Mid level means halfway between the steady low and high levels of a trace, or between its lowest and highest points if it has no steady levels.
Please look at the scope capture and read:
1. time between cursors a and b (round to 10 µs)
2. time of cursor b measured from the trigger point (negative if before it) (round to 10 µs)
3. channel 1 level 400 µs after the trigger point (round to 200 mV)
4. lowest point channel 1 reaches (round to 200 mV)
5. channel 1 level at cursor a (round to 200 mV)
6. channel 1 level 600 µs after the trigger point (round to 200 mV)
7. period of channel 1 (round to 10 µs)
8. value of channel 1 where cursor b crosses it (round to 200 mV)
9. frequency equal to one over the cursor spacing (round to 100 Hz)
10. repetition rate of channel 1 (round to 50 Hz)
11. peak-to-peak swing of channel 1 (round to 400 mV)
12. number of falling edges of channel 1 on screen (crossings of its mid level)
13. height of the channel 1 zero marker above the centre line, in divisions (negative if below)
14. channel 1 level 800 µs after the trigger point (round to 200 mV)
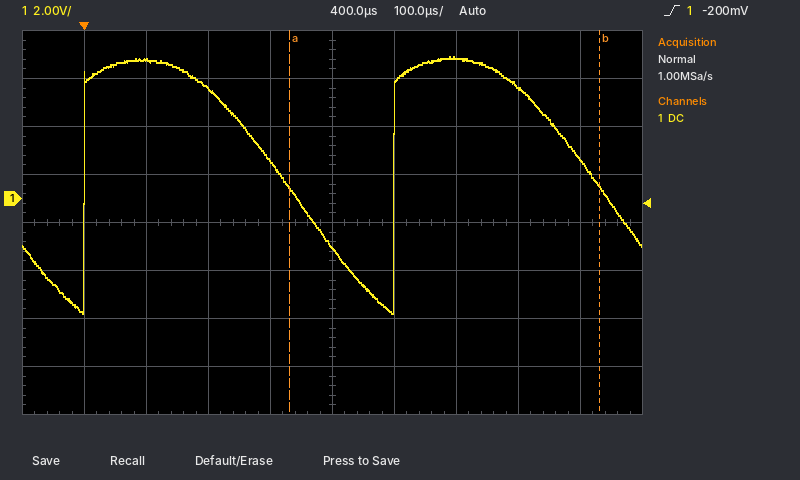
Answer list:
500 µs
+830 µs
-2.0 V
-4.8 V
400 mV
5.8 V
500 µs
600 mV
2.0 kHz
2.00 kHz
10.8 V
2
+0.5 div
1.6 V
